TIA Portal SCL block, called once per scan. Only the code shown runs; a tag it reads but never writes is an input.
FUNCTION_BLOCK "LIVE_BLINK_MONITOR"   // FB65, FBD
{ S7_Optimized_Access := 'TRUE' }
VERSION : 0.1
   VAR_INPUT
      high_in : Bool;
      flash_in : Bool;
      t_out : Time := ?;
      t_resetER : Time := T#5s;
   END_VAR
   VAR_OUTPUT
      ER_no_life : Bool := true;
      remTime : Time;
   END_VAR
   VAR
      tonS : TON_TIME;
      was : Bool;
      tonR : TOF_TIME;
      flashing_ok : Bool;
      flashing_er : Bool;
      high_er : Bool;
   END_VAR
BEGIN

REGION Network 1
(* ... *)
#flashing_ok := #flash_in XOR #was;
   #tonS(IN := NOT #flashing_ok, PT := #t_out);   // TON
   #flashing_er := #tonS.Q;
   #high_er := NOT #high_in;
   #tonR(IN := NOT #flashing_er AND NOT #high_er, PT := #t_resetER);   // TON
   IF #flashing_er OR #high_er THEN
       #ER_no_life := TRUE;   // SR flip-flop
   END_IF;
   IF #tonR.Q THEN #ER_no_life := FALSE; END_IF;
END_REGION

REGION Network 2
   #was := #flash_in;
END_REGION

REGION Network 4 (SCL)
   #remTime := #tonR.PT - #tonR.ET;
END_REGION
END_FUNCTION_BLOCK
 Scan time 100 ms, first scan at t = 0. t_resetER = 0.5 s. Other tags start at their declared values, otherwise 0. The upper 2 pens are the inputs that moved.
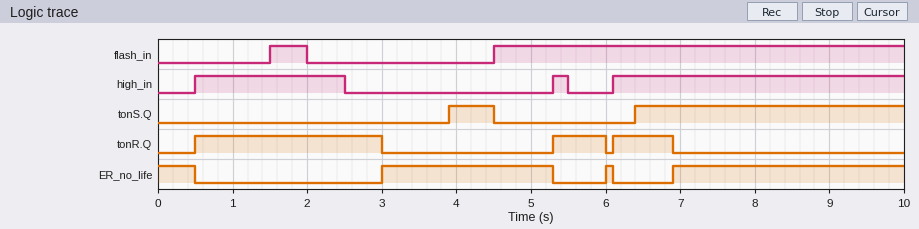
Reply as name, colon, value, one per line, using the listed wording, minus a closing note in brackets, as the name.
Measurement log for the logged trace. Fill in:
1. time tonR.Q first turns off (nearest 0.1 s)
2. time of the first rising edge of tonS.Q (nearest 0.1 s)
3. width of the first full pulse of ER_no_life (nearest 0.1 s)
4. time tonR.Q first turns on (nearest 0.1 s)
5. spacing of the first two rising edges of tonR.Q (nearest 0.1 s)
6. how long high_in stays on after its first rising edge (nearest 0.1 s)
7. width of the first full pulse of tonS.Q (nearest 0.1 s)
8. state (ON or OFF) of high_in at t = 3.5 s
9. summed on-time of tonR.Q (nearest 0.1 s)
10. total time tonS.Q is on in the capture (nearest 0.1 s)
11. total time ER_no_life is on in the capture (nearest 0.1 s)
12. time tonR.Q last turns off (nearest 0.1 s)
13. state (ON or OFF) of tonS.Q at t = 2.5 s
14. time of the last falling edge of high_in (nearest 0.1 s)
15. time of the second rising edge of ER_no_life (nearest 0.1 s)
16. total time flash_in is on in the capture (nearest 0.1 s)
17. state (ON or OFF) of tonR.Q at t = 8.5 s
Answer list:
time tonR.Q first turns off: 3.0 s
time of the first rising edge of tonS.Q: 3.9 s
width of the first full pulse of ER_no_life: 2.3 s
time tonR.Q first turns on: 0.5 s
spacing of the first two rising edges of tonR.Q: 4.8 s
how long high_in stays on after its first rising edge: 2.0 s
width of the first full pulse of tonS.Q: 0.6 s
state (ON or OFF) of high_in at t = 3.5 s: OFF
summed on-time of tonR.Q: 4.0 s
total time tonS.Q is on in the capture: 4.2 s
total time ER_no_life is on in the capture: 6.0 s
time tonR.Q last turns off: 6.9 s
state (ON or OFF) of tonS.Q at t = 2.5 s: OFF
time of the last falling edge of high_in: 5.5 s
time of the second rising edge of ER_no_life: 6.0 s
total time flash_in is on in the capture: 6.0 s
state (ON or OFF) of tonR.Q at t = 8.5 s: OFF
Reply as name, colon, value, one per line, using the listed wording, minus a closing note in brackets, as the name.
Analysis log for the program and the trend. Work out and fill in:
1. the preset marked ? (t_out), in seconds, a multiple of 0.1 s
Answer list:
the preset marked ? (t_out), in seconds, a multiple of 0.1 s: 1.8 s
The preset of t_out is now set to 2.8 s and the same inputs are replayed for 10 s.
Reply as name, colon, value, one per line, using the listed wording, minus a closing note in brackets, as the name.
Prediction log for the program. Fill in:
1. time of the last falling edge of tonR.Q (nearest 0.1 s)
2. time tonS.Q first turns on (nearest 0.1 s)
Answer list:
time of the last falling edge of tonR.Q: 7.9 s
time tonS.Q first turns on: 7.4 s
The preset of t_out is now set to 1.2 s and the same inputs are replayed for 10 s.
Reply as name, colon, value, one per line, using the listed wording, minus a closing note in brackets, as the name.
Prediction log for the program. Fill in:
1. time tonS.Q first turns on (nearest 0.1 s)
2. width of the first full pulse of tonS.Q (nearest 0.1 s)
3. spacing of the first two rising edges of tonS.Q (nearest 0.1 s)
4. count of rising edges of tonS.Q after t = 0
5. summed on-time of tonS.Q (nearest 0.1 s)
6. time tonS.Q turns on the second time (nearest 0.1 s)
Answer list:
time tonS.Q first turns on: 1.2 s
width of the first full pulse of tonS.Q: 0.3 s
spacing of the first two rising edges of tonS.Q: 2.1 s
count of rising edges of tonS.Q after t = 0: 3
summed on-time of tonS.Q: 5.7 s
time tonS.Q turns on the second time: 3.3 s
